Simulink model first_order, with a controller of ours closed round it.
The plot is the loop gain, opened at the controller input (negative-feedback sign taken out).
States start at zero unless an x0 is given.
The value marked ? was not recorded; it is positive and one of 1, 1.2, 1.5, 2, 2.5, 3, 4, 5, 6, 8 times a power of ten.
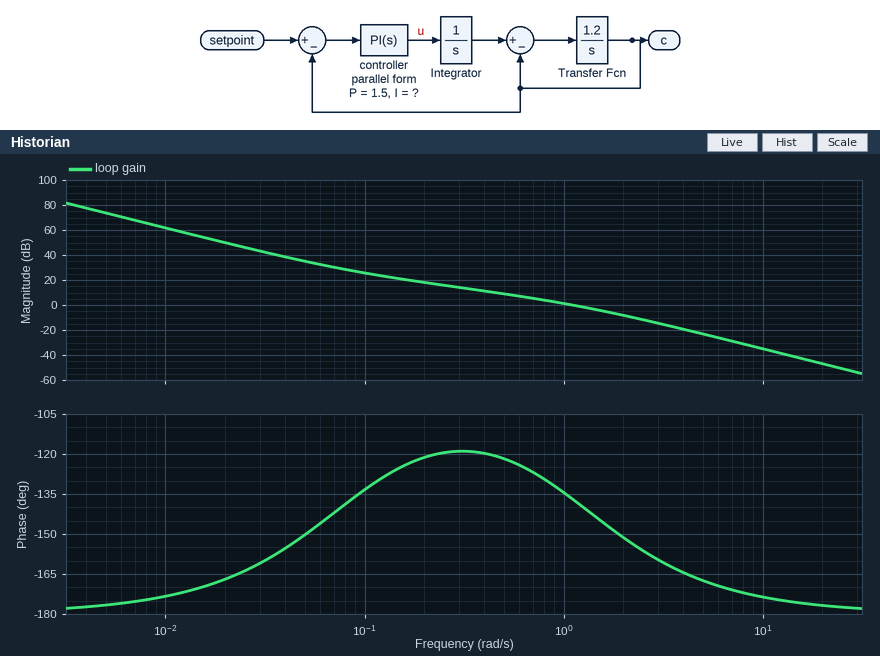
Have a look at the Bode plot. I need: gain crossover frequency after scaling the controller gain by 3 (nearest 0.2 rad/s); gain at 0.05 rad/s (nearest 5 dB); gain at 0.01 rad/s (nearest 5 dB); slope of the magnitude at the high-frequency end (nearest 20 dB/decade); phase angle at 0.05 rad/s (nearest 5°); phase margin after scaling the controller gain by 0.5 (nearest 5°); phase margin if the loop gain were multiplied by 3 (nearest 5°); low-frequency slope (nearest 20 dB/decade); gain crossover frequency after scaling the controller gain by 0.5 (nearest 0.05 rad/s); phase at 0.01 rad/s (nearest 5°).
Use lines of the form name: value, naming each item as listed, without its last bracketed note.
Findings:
gain crossover frequency after scaling the controller gain by 3: 2.2 rad/s
gain at 0.05 rad/s: 35 dB
gain at 0.01 rad/s: 60 dB
slope of the magnitude at the high-frequency end: -40 dB/decade
phase angle at 0.05 rad/s: -150°
phase margin after scaling the controller gain by 0.5: 55°
phase margin if the loop gain were multiplied by 3: 25°
low-frequency slope: -40 dB/decade
gain crossover frequency after scaling the controller gain by 0.5: 0.65 rad/s
phase at 0.01 rad/s: -175°
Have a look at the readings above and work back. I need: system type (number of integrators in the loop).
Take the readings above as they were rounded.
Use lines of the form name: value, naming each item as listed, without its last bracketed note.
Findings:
system type: 2
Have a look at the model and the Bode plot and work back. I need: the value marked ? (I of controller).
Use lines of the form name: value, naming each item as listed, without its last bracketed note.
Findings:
the value marked ?: 0.12
